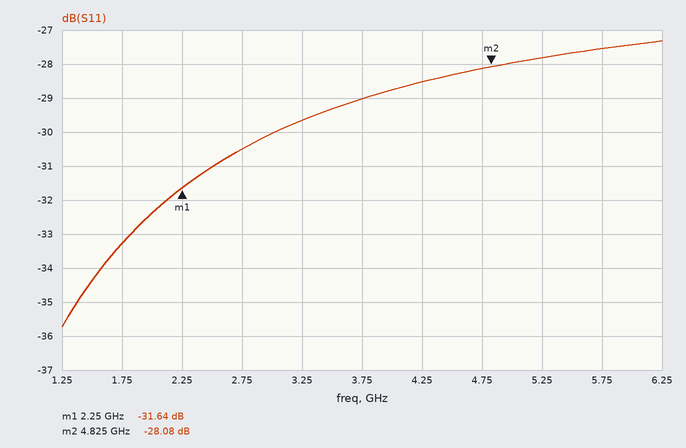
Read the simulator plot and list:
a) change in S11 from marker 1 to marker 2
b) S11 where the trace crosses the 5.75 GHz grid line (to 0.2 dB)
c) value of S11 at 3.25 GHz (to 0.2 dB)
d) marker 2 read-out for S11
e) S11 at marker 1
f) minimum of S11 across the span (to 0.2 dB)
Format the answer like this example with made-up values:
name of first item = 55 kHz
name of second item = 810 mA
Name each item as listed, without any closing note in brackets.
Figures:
change in S11 from marker 1 to marker 2 = 3.56 dB
S11 where the trace crosses the 5.75 GHz grid line = -27.6 dB
value of S11 at 3.25 GHz = -29.6 dB
marker 2 read-out for S11 = -28.08 dB
S11 at marker 1 = -31.64 dB
minimum of S11 across the span = -35.8 dB
